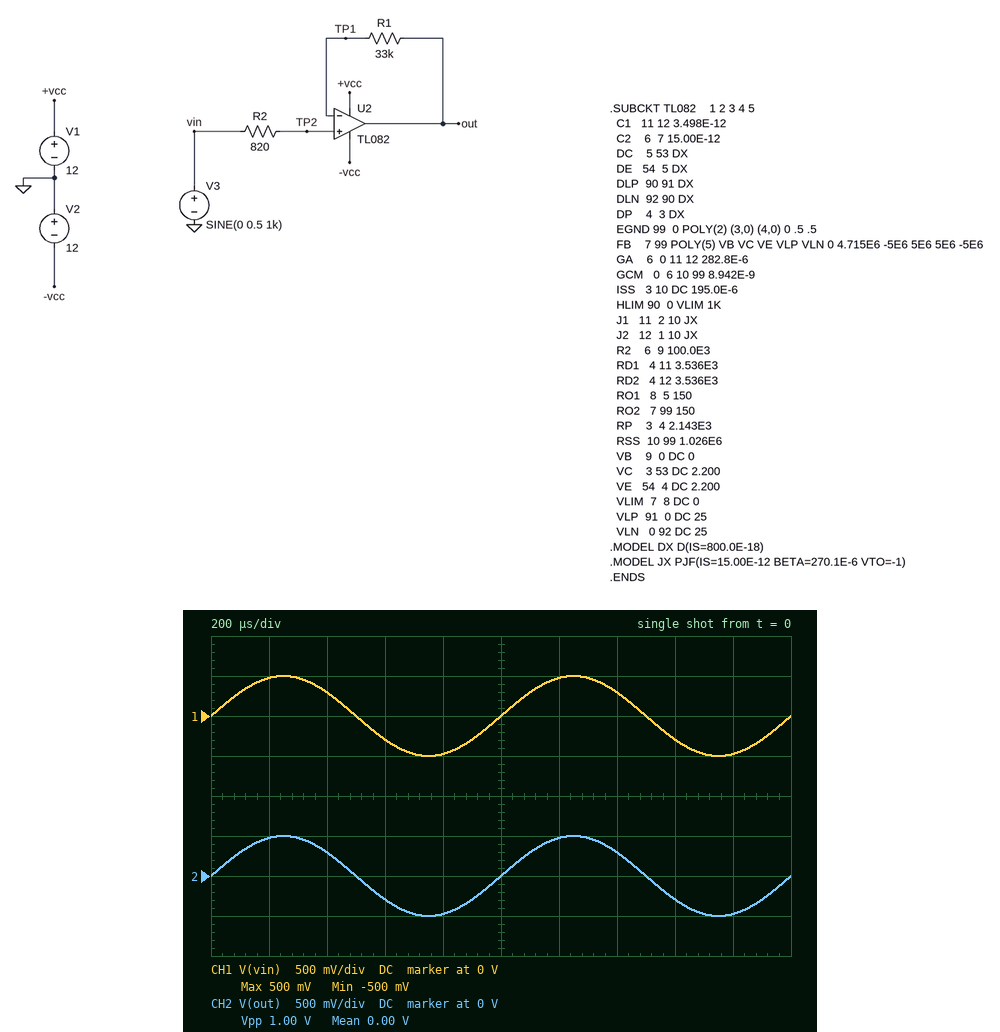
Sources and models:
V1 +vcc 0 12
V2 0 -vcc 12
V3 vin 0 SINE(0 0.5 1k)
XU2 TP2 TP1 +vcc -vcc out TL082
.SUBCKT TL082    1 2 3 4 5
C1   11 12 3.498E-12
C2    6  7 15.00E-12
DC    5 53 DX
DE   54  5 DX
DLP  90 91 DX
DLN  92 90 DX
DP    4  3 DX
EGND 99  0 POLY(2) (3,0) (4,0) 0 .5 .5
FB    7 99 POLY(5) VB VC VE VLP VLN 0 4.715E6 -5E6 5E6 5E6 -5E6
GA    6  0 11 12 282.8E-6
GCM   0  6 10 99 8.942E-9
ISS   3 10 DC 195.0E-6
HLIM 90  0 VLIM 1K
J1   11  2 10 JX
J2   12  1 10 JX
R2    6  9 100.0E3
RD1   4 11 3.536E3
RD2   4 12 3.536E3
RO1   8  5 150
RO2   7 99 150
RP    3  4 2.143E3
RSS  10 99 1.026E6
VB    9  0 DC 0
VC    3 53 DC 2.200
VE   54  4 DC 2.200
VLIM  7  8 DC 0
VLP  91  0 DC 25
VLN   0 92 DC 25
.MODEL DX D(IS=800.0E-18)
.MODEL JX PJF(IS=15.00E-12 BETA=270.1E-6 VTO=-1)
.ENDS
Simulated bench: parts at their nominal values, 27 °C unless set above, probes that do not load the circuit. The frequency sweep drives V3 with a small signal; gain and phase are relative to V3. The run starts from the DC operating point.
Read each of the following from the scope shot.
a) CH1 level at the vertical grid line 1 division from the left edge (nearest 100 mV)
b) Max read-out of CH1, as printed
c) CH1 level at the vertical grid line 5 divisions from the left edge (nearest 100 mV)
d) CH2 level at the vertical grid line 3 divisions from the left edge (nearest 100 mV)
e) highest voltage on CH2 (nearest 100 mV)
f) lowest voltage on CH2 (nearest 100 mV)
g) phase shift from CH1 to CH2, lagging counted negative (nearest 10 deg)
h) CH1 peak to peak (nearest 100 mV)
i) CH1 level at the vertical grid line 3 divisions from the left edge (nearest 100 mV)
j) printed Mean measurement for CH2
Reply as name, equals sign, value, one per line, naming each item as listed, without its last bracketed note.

CH1 level at the vertical grid line 1 division from the left edge = 500 mV
Max read-out of CH1, as printed = 500 mV
CH1 level at the vertical grid line 5 divisions from the left edge = 0 V
CH2 level at the vertical grid line 3 divisions from the left edge = -300 mV
highest voltage on CH2 = 500 mV
lowest voltage on CH2 = -500 mV
phase shift from CH1 to CH2, lagging counted negative = 0 deg
CH1 peak to peak = 1.0 V
CH1 level at the vertical grid line 3 divisions from the left edge = -300 mV
printed Mean measurement for CH2 = 0.00 V
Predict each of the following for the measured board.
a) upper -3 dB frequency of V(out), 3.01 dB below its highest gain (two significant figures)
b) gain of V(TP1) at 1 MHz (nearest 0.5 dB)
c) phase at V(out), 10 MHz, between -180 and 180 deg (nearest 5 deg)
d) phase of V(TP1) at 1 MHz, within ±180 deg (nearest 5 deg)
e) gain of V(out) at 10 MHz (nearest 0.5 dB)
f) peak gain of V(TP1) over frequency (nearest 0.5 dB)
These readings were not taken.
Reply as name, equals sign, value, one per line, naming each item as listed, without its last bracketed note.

upper -3 dB frequency of V(out), 3.01 dB below its highest gain = 4.9 MHz
gain of V(TP1) at 1 MHz = 0 dB
phase at V(out), 10 MHz, between -180 and 180 deg = -140 deg
phase of V(TP1) at 1 MHz, within ±180 deg = -15 deg
gain of V(out) at 10 MHz = -13.0 dB
peak gain of V(TP1) over frequency = 0 dB
